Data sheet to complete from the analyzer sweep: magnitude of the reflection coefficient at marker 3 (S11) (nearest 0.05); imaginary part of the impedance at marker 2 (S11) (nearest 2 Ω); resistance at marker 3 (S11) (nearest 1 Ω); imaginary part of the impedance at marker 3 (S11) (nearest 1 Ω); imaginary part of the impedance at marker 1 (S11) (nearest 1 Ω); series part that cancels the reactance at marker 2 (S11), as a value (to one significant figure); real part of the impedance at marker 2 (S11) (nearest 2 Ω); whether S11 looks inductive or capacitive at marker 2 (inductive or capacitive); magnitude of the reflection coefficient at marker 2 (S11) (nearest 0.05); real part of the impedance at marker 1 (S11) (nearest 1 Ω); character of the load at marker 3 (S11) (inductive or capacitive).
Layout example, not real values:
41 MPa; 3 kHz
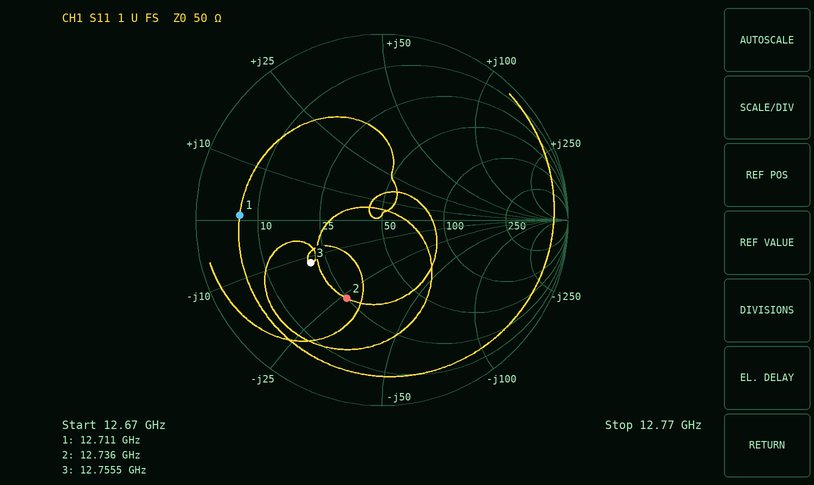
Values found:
0.45; -26 Ω; 20 Ω; -12 Ω; +1 Ω; 300 pH; 24 Ω; capacitive; 0.45; 7 Ω; capacitive
